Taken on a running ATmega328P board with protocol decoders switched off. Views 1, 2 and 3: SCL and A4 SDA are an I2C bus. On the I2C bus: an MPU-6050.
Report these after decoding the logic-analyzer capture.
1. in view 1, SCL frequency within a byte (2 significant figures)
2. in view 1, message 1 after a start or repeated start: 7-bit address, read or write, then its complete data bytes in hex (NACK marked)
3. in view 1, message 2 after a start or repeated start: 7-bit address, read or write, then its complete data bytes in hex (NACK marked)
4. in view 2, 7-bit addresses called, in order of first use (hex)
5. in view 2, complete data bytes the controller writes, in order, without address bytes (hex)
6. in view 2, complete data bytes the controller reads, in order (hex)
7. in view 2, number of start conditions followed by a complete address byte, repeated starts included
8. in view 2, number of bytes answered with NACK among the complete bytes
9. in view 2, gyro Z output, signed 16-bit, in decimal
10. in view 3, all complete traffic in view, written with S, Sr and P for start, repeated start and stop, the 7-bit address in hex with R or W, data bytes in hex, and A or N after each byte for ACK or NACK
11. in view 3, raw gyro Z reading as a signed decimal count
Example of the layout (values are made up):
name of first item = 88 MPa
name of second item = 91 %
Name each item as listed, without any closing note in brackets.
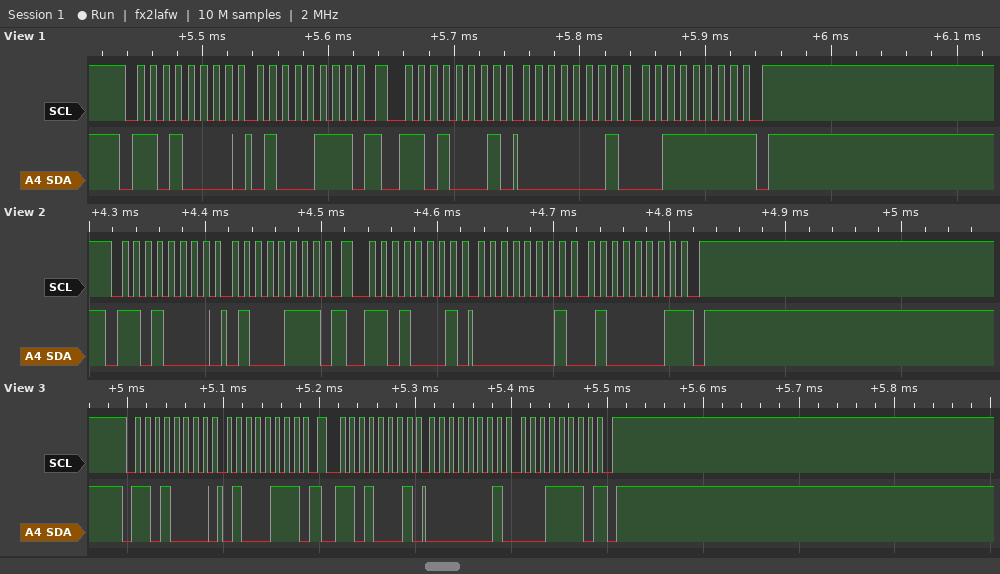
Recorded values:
in view 1, SCL frequency within a byte = 100 kHz
in view 1, message 1 after a start or repeated start: 7-bit address, read or write, then its complete data bytes in hex = 0x68 write: 47
in view 1, message 2 after a start or repeated start: 7-bit address, read or write, then its complete data bytes in hex = 0x68 read: 01 3F NACK
in view 2, 7-bit addresses called, in order of first use = 0x68
in view 2, complete data bytes the controller writes, in order, without address bytes = 47
in view 2, complete data bytes the controller reads, in order = 01 41
in view 2, number of start conditions followed by a complete address byte, repeated starts included = 2
in view 2, number of bytes answered with NACK among the complete bytes = 1
in view 2, gyro Z output, signed 16-bit, in decimal = 321
in view 3, all complete traffic in view, written with S, Sr and P for start, repeated start and stop, the 7-bit address in hex with R or W, data bytes in hex, and A or N after each byte for ACK or NACK = S 68W A 47 A Sr 68R A 01 A 1E N P
in view 3, raw gyro Z reading as a signed decimal count = 286
